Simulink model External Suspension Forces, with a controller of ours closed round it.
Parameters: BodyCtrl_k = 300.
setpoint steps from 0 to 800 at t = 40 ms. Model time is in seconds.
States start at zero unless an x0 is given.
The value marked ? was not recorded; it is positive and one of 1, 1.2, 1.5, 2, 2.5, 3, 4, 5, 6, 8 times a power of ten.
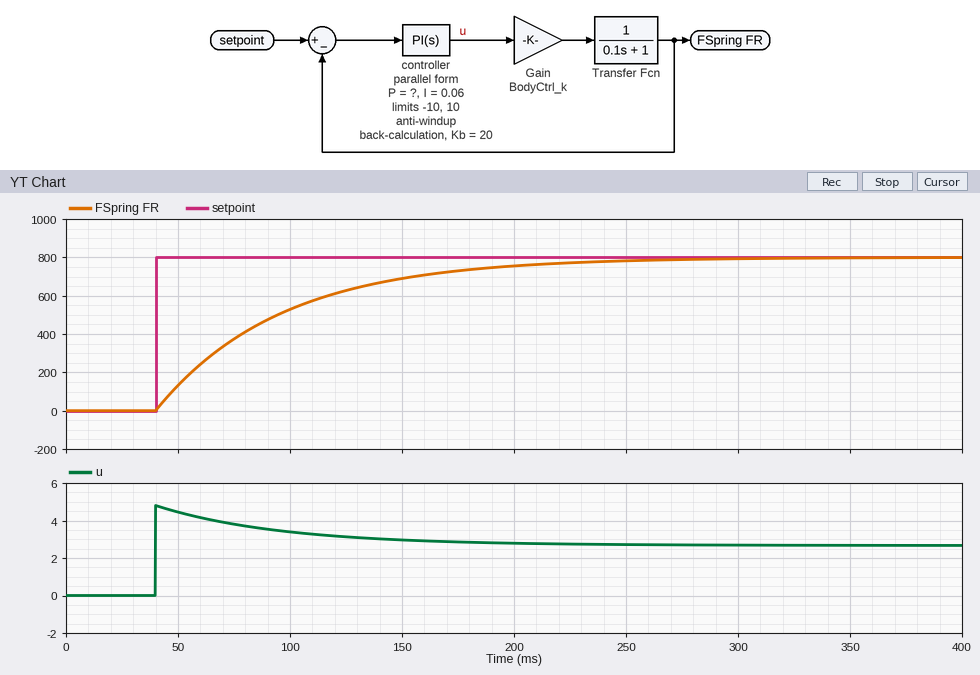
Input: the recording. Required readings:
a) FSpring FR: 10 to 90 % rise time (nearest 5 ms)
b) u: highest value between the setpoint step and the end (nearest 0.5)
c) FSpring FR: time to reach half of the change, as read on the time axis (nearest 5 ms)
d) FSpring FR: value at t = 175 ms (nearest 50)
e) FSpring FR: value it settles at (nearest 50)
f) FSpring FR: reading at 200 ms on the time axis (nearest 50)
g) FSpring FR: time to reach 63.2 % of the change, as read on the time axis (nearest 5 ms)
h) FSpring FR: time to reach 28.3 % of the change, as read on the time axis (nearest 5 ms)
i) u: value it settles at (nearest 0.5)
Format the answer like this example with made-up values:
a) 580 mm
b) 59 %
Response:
a) 120 ms
b) 5.0
c) 80 ms
d) 750
e) 800
f) 750
g) 95 ms
h) 60 ms
i) 2.5
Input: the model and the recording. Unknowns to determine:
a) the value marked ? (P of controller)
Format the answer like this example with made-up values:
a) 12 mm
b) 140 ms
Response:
a) 0.006
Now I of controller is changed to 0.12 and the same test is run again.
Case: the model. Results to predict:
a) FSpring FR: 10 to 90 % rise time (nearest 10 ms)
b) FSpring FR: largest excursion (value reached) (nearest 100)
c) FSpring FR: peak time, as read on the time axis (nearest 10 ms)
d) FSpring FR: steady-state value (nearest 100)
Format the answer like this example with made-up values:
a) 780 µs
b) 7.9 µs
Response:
a) 70 ms
b) 900
c) 200 ms
d) 800
